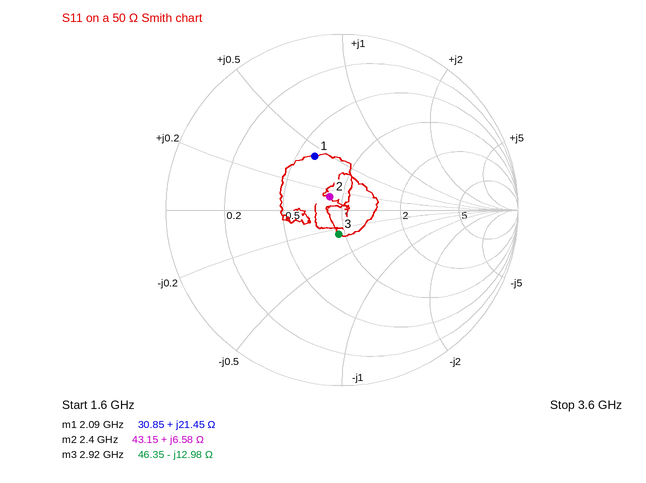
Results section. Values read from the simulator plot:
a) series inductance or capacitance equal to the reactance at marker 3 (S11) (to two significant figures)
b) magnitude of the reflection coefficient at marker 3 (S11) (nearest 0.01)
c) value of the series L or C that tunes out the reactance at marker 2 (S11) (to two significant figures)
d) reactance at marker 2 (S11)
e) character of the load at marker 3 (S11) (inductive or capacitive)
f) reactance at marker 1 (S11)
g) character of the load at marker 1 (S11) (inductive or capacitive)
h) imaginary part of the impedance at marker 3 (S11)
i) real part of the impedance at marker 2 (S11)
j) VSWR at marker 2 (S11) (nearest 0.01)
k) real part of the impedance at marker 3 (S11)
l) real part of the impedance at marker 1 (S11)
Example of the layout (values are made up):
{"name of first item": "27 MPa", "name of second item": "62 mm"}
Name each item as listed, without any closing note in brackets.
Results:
{"series inductance or capacitance equal to the reactance at marker 3 (S11)": "4.2 pF", "magnitude of the reflection coefficient at marker 3 (S11)": "0.14", "value of the series L or C that tunes out the reactance at marker 2 (S11)": "10 pF", "reactance at marker 2": "+6.58 Ω", "character of the load at marker 3 (S11)": "capacitive", "reactance at marker 1": "+21.45 Ω", "character of the load at marker 1 (S11)": "inductive", "imaginary part of the impedance at marker 3": "-12.98 Ω", "real part of the impedance at marker 2": "43.15 Ω", "VSWR at marker 2 (S11)": "1.23", "real part of the impedance at marker 3": "46.35 Ω", "real part of the impedance at marker 1": "30.85 Ω"}
